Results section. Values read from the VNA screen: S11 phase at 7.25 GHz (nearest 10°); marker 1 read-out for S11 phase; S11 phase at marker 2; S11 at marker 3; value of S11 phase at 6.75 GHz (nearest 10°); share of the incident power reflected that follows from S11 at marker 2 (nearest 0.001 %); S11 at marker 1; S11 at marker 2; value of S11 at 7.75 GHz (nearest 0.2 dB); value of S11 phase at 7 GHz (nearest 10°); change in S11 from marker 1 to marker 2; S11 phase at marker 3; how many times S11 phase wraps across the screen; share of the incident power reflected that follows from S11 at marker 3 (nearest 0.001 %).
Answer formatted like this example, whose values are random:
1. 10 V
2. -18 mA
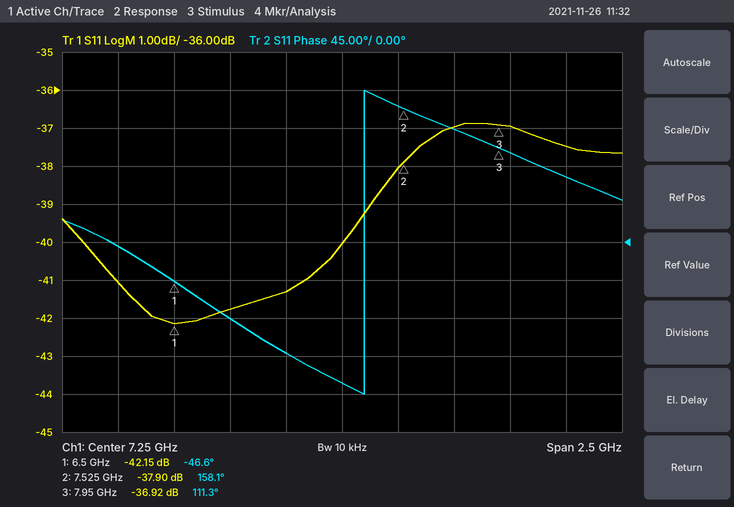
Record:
1. -170°
2. -46.6°
3. 158.1°
4. -36.92 dB
5. -90°
6. 0.016 %
7. -42.15 dB
8. -37.90 dB
9. -37.0 dB
10. -130°
11. 4.25 dB
12. 111.3°
13. 1
14. 0.020 %
